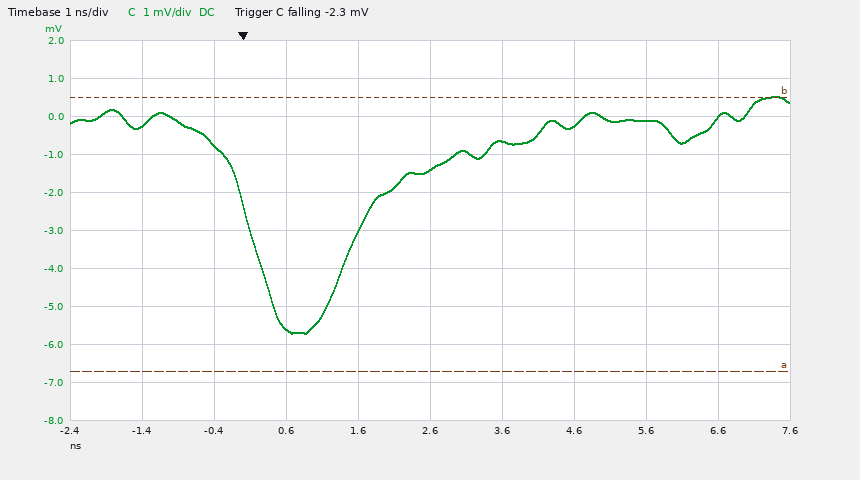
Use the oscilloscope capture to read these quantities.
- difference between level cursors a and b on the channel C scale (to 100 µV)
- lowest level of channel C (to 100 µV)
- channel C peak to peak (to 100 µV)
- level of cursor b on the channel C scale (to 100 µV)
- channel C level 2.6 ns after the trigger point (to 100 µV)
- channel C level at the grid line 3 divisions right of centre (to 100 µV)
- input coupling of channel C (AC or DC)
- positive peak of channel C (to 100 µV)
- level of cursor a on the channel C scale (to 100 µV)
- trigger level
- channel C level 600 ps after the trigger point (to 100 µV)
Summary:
7.2 mV
-5.7 mV
6.2 mV
500 µV
-1.4 mV
-100 µV
DC
500 µV
-6.7 mV
-2.3 mV
-5.6 mV
